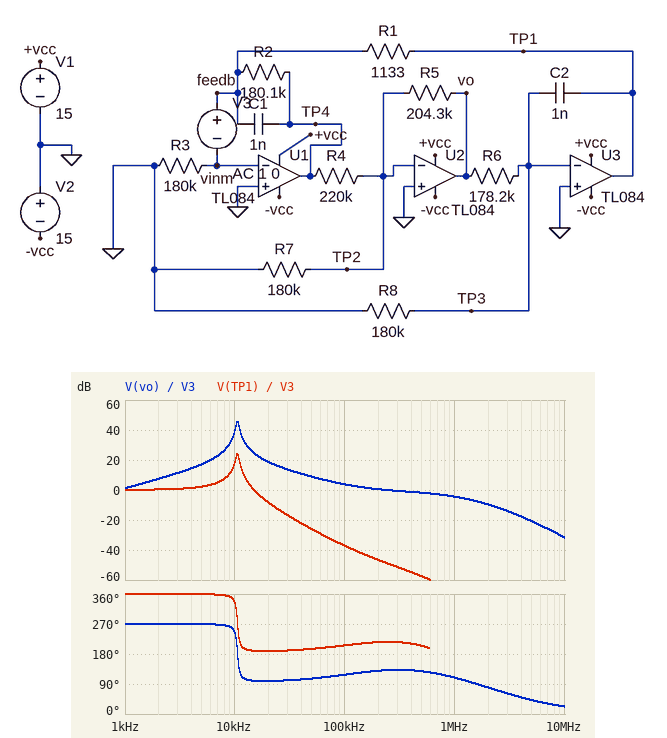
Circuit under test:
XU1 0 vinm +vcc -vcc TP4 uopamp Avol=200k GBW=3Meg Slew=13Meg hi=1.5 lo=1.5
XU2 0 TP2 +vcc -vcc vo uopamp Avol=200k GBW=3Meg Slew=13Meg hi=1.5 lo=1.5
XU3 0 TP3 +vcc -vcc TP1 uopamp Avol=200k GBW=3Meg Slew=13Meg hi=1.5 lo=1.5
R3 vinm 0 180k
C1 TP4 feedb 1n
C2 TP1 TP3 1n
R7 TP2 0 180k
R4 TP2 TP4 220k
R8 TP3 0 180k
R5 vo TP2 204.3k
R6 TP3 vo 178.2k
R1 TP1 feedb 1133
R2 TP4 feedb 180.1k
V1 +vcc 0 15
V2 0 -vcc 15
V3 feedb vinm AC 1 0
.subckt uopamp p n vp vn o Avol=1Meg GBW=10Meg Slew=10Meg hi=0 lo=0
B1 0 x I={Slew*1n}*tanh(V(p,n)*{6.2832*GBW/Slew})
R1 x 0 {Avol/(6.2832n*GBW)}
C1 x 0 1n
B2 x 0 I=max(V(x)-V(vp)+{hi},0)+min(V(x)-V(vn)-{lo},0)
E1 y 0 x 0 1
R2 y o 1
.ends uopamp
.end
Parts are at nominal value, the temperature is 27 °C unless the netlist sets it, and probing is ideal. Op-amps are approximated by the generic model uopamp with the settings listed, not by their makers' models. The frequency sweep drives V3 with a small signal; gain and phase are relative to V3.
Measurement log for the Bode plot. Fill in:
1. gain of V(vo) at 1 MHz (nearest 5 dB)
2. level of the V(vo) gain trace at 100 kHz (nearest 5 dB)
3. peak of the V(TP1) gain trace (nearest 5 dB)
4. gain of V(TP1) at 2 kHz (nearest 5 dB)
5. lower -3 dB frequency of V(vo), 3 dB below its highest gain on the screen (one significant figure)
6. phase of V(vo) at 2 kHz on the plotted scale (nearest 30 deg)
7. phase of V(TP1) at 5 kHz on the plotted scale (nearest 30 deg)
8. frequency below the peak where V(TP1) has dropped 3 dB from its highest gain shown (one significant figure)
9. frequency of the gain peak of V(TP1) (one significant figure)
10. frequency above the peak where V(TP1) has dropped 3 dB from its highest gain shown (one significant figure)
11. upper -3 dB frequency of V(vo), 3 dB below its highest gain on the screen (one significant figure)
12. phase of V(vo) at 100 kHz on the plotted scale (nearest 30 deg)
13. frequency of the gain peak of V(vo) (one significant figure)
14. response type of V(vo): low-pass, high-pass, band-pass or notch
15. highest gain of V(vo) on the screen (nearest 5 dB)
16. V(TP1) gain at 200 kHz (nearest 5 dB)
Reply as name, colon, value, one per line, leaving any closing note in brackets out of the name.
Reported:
gain of V(vo) at 1 MHz: -5 dB
level of the V(vo) gain trace at 100 kHz: 5 dB
peak of the V(TP1) gain trace: 25 dB
gain of V(TP1) at 2 kHz: 0 dB
lower -3 dB frequency of V(vo), 3 dB below its highest gain on the screen: 10 kHz
phase of V(vo) at 2 kHz on the plotted scale: 270 deg
phase of V(TP1) at 5 kHz on the plotted scale: 360 deg
frequency below the peak where V(TP1) has dropped 3 dB from its highest gain shown: 10 kHz
frequency of the gain peak of V(TP1): 10 kHz
frequency above the peak where V(TP1) has dropped 3 dB from its highest gain shown: 10 kHz
upper -3 dB frequency of V(vo), 3 dB below its highest gain on the screen: 10 kHz
phase of V(vo) at 100 kHz on the plotted scale: 120 deg
frequency of the gain peak of V(vo): 10 kHz
response type of V(vo): low-pass, high-pass, band-pass or notch: band-pass
highest gain of V(vo) on the screen: 45 dB
V(TP1) gain at 200 kHz: -45 dB
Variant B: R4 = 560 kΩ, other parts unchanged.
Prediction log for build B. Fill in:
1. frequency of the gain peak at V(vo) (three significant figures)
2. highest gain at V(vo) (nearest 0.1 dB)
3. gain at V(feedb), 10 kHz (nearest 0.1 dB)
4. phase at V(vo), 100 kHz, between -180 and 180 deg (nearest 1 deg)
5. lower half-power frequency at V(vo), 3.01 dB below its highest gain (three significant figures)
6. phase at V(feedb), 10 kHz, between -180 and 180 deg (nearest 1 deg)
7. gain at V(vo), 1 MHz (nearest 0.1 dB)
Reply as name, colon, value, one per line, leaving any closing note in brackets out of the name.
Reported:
frequency of the gain peak at V(vo): 6.61 kHz
highest gain at V(vo): 36.0 dB
gain at V(feedb), 10 kHz: -0.7 dB
phase at V(vo), 100 kHz, between -180 and 180 deg: 119 deg
lower half-power frequency at V(vo), 3.01 dB below its highest gain: 6.23 kHz
phase at V(feedb), 10 kHz, between -180 and 180 deg: -1 deg
gain at V(vo), 1 MHz: -11.8 dB
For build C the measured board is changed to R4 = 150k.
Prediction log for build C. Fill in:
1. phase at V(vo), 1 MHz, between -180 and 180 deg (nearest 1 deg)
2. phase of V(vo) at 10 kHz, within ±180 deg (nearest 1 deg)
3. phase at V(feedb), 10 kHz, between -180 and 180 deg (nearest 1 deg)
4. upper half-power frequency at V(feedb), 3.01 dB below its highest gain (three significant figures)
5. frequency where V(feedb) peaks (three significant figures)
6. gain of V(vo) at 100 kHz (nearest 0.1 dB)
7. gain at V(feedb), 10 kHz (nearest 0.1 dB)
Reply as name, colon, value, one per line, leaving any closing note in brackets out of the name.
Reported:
phase at V(vo), 1 MHz, between -180 and 180 deg: 105 deg
phase of V(vo) at 10 kHz, within ±180 deg: -92 deg
phase at V(feedb), 10 kHz, between -180 and 180 deg: 0 deg
upper half-power frequency at V(feedb), 3.01 dB below its highest gain: 12.9 kHz
frequency where V(feedb) peaks: 12.6 kHz
gain of V(vo) at 100 kHz: 7.1 dB
gain at V(feedb), 10 kHz: 0.6 dB
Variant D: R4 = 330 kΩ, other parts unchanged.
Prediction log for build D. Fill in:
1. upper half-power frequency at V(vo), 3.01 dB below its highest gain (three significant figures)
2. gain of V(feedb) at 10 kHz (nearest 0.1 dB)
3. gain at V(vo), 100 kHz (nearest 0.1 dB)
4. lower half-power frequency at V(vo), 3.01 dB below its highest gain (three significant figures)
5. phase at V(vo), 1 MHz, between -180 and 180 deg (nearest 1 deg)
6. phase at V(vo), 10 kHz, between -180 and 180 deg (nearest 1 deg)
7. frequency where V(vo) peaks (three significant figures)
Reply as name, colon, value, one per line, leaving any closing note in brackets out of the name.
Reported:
upper half-power frequency at V(vo), 3.01 dB below its highest gain: 8.98 kHz
gain of V(feedb) at 10 kHz: -1.5 dB
gain at V(vo), 100 kHz: 0.2 dB
lower half-power frequency at V(vo), 3.01 dB below its highest gain: 8.25 kHz
phase at V(vo), 1 MHz, between -180 and 180 deg: 112 deg
phase at V(vo), 10 kHz, between -180 and 180 deg: 109 deg
frequency where V(vo) peaks: 8.61 kHz
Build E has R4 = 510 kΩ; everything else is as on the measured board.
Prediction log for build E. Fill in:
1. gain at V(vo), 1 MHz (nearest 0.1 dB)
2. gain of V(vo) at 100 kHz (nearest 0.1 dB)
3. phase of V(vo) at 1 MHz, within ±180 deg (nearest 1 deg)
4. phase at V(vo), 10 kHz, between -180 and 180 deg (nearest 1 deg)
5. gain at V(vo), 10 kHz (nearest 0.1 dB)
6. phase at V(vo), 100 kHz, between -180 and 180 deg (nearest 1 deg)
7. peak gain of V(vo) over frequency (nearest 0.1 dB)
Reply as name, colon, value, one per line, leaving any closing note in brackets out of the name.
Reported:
gain at V(vo), 1 MHz: -11.0 dB
gain of V(vo) at 100 kHz: -3.6 dB
phase of V(vo) at 1 MHz, within ±180 deg: 114 deg
phase at V(vo), 10 kHz, between -180 and 180 deg: 102 deg
gain at V(vo), 10 kHz: 20.3 dB
phase at V(vo), 100 kHz, between -180 and 180 deg: 119 deg
peak gain of V(vo) over frequency: 36.9 dB
